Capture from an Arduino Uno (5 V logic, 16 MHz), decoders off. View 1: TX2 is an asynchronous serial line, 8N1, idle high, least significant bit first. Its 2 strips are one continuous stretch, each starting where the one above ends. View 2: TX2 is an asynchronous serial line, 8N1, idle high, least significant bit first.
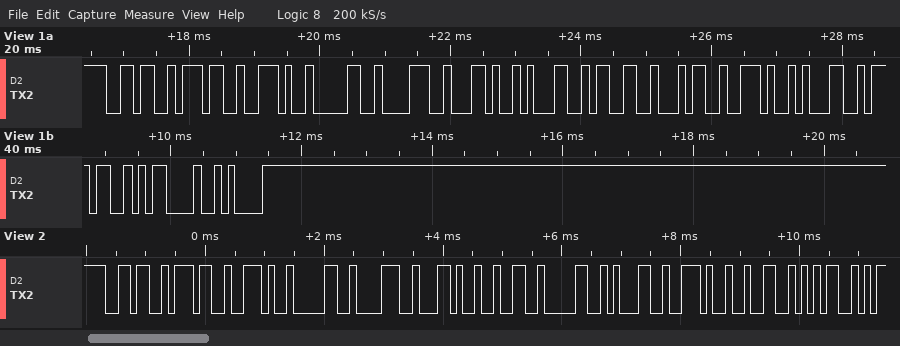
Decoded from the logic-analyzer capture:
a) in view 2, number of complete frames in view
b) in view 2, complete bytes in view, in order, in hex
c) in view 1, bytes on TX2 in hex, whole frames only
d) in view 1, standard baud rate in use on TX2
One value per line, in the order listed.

12
36 37 2E 30 38 2C 32 30 31 2E 32 35
36 37 2E 30 38 2C 31 33 34 2E 31 37 0D 0A
9600 baud
